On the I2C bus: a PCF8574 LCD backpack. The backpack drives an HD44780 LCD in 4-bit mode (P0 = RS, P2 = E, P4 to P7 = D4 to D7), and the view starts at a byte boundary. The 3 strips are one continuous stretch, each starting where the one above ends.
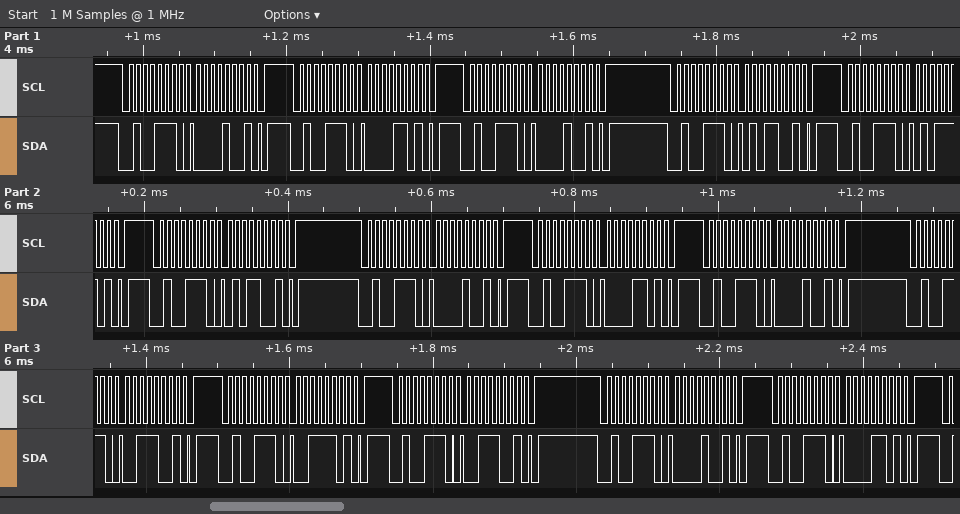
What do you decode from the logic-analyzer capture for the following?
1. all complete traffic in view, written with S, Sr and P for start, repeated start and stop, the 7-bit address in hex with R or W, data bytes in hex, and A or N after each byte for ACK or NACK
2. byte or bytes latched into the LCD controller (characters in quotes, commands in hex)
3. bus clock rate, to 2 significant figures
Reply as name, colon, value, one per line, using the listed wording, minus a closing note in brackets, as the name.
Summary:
all complete traffic in view, written with S, Sr and P for start, repeated start and stop, the 7-bit address in hex with R or W, data bytes in hex, and A or N after each byte for ACK or NACK: S 27W A 09 A P S 27W A 0D A P S 27W A 09 A P S 27W A 59 A P S 27W A 5D A P S 27W A 59 A P S 27W A 09 A P S 27W A 0D A P S 27W A 09 A P S 27W A 39 A P S 27W A 3D A P S 27W A 39 A P S 27W A 09 A P S 27W A 0D A P
byte or bytes latched into the LCD controller: data 0x05 data 0x03
bus clock rate, to 2 significant figures: 100 kHz
